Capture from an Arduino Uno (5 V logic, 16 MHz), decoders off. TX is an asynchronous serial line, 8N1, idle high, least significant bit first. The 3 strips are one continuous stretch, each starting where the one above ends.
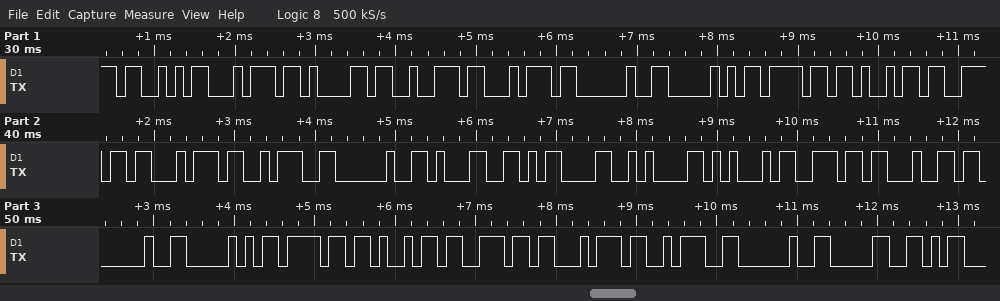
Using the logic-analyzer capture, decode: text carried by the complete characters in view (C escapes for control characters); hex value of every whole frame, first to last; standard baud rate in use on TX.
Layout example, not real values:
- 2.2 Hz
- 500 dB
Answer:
- "Start Point: 1\r\nEnd Point: 0"
- 0x53 0x74 0x61 0x72 0x74 0x20 0x50 0x6F 0x69 0x6E 0x74 0x3A 0x20 0x31 0x0D 0x0A 0x45 0x6E 0x64 0x20 0x50 0x6F 0x69 0x6E 0x74 0x3A 0x20 0x30
- 9600 baud
